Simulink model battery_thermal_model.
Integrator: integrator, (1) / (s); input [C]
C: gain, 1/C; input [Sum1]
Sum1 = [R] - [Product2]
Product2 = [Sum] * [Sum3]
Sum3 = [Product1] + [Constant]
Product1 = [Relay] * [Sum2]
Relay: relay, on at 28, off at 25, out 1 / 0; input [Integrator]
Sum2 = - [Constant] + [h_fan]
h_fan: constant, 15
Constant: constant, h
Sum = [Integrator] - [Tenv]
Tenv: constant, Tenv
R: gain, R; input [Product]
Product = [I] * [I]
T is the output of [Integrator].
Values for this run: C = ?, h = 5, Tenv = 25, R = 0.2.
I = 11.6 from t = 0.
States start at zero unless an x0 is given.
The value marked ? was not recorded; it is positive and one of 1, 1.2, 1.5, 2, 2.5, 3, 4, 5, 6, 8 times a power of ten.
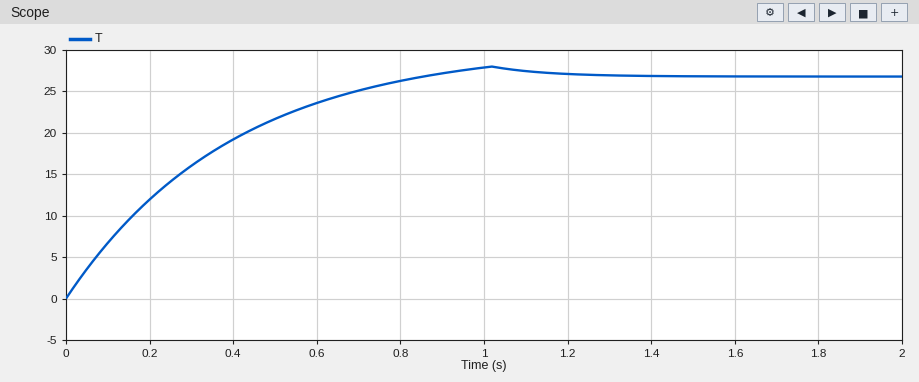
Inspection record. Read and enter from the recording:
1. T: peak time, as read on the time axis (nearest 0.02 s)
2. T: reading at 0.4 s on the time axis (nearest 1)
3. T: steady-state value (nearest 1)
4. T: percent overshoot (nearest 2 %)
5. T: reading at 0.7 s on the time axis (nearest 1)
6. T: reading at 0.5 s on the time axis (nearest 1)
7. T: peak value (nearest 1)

1.02 s
19
27
4 %
25
22
28
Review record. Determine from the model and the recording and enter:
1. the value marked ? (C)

2
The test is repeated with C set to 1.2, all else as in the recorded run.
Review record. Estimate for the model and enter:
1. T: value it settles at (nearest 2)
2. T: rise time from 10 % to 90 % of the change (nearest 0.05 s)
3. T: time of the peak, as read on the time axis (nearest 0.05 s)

26
0.35 s
0.60 s
